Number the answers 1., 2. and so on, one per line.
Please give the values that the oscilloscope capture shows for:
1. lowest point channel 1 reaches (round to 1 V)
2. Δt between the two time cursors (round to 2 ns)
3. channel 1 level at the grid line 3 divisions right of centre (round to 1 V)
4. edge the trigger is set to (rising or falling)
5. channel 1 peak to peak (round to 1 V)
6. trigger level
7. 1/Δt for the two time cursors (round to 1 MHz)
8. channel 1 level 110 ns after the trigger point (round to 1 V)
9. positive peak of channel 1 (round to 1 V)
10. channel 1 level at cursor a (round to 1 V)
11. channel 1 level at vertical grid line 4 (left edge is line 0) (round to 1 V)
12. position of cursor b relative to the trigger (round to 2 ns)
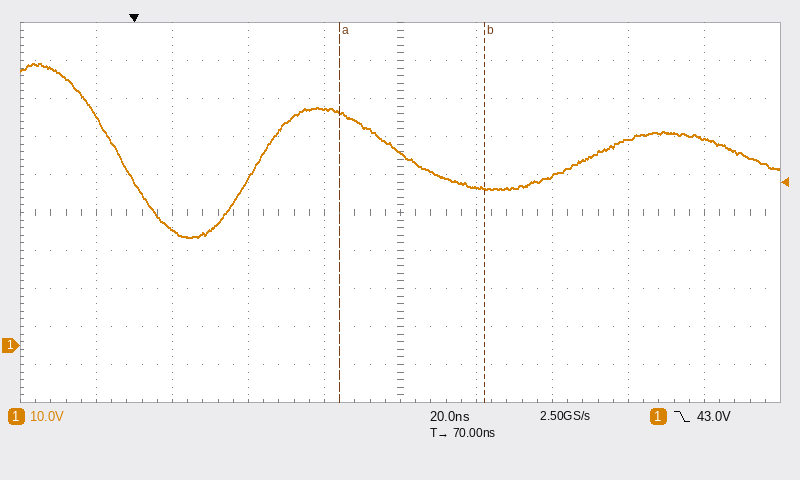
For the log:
1. 28 V
2. 38 ns
3. 54 V
4. falling
5. 46 V
6. 43.0 V
7. 26 MHz
8. 45 V
9. 74 V
10. 61 V
11. 62 V
12. +92 ns
